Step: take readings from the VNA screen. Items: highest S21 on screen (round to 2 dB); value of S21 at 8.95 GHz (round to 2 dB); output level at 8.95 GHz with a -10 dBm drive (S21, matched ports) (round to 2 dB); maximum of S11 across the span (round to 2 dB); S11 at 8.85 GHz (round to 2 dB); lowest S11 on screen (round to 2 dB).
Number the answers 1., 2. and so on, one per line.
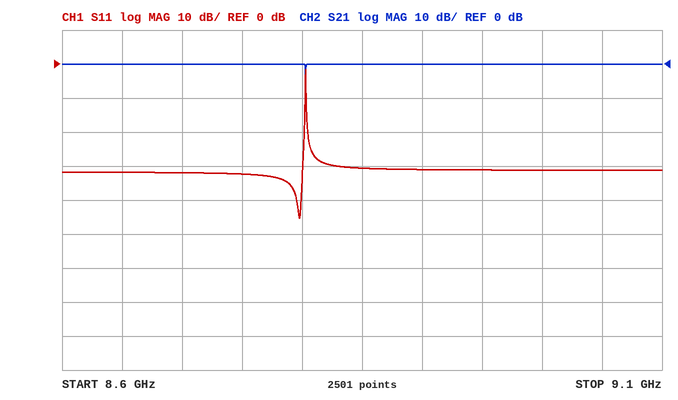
1. 0 dB
2. 0 dB
3. -10 dBm
4. -2 dB
5. -30 dB
6. -46 dB
